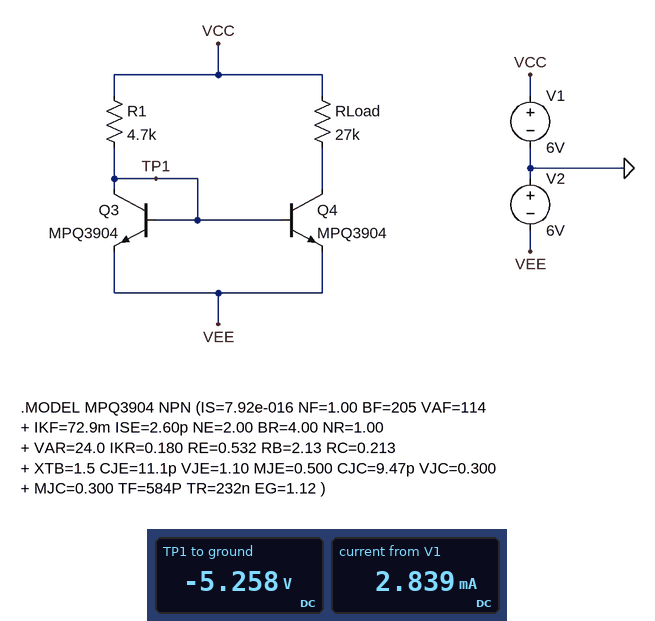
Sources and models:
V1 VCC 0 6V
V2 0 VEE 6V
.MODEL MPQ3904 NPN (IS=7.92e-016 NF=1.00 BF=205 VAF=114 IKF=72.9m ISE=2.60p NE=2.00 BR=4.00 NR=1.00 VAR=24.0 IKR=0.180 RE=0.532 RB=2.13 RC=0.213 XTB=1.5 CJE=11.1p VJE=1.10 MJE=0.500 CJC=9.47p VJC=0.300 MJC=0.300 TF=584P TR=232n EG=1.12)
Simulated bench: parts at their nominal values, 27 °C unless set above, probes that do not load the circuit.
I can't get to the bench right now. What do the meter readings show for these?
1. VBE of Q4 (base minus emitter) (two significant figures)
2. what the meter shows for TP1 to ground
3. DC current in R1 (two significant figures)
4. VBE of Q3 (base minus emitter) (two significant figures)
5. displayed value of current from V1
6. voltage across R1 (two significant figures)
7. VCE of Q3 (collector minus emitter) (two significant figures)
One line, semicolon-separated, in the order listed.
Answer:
740 mV; -5.258 V; 2.4 mA; 740 mV; 2.839 mA; 11 V; 740 mV
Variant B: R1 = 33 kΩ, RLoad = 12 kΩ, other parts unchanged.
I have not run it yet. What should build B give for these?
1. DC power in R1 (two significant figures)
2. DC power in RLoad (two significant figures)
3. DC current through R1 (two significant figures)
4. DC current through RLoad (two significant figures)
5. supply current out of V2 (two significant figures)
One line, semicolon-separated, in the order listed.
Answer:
3.9 mW; 1.5 mW; 340 µA; 360 µA; 700 µA
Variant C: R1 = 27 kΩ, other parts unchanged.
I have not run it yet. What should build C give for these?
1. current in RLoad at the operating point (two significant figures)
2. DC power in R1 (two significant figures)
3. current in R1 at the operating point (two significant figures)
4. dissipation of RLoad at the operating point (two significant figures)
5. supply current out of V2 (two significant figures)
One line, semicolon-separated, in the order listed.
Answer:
410 µA; 4.7 mW; 420 µA; 4.6 mW; 830 µA
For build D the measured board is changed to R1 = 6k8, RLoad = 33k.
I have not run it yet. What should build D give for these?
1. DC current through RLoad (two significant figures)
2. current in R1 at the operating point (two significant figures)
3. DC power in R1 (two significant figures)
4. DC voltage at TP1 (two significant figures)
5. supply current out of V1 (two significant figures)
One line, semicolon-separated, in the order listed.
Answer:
360 µA; 1.7 mA; 19 mW; -5.3 V; 2.0 mA
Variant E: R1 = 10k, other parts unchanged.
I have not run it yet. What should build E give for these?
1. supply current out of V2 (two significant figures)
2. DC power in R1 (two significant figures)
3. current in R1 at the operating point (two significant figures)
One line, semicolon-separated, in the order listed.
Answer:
1.6 mA; 13 mW; 1.1 mA
